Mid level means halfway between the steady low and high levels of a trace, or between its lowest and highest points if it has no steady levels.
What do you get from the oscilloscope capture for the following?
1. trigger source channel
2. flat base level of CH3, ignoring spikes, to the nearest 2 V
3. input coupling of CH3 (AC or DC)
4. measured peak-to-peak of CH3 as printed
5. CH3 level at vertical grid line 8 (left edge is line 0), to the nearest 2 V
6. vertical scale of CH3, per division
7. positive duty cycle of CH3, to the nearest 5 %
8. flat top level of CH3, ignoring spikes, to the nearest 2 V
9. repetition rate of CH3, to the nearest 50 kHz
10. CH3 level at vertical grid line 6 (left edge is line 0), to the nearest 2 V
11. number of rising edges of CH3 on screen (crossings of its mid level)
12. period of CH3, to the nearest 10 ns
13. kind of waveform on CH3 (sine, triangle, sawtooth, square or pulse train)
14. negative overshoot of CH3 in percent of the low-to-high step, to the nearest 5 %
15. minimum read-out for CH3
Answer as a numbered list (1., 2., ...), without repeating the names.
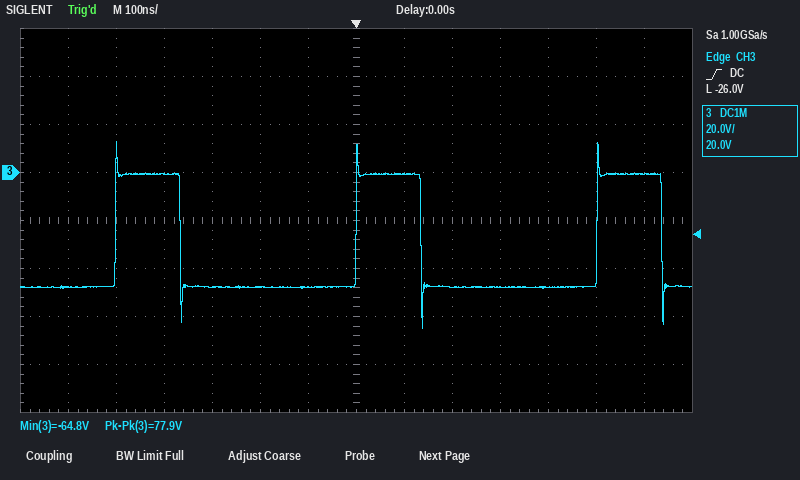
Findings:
1. CH3
2. -48 V
3. DC
4. 77.9 V
5. 0 V
6. 20 V
7. 25 %
8. 0 V
9. 2.00 MHz
10. -48 V
11. 3
12. 500 ns
13. pulse train
14. 35 %
15. -64.8 V
